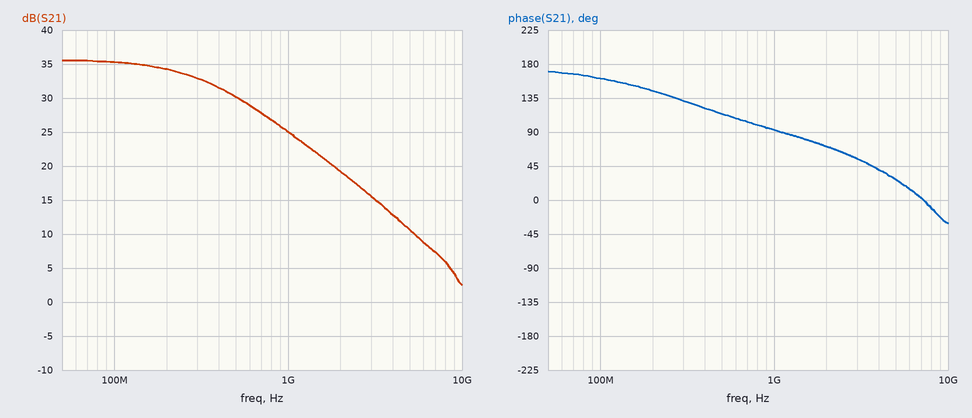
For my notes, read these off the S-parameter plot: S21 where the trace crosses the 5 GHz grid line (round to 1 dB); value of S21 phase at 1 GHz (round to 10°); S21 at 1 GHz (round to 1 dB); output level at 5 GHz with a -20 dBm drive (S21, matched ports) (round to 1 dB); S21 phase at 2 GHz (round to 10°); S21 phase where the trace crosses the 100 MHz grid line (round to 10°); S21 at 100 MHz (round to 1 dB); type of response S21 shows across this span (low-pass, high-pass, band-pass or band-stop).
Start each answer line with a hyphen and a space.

- 11 dB
- 90°
- 25 dB
- -9 dBm
- 70°
- 160°
- 35 dB
- low-pass
